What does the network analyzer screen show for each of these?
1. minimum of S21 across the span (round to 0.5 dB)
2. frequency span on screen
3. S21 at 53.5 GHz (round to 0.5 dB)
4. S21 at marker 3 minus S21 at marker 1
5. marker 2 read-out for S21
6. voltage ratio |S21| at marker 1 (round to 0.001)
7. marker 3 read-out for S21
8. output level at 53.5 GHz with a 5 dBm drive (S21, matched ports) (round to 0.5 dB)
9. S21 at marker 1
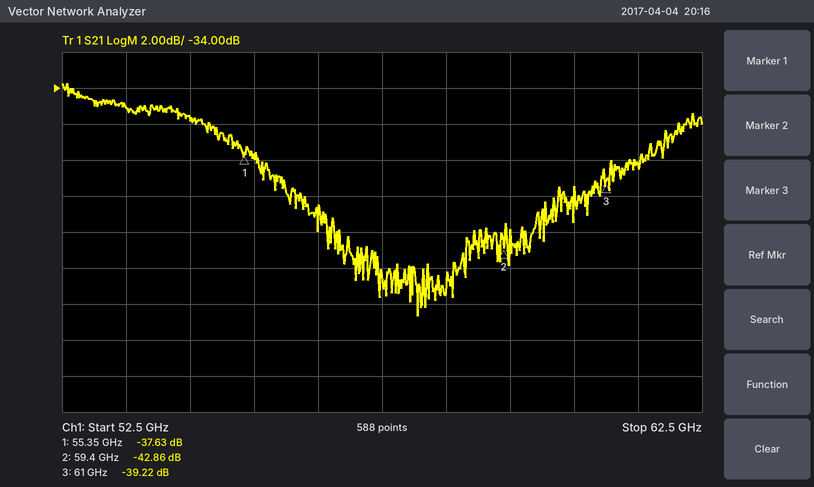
-46.5 dB
10 GHz
-35.0 dB
-1.59 dB
-42.86 dB
0.013
-39.22 dB
-30.0 dBm
-37.63 dB
